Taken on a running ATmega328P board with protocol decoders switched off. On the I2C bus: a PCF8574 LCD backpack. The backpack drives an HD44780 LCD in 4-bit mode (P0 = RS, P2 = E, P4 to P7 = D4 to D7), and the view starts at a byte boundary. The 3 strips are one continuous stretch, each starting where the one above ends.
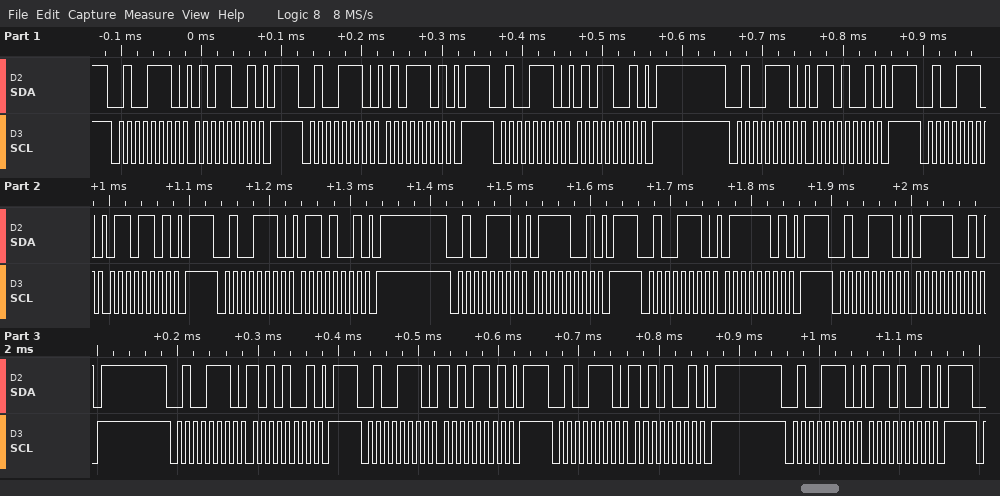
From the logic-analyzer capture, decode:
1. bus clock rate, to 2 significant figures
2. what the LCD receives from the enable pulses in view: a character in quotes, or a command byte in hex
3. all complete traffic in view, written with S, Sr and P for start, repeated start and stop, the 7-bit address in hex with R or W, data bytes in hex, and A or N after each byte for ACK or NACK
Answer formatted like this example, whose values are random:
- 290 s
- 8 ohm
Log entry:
- 100 kHz
- 'V' 'z'
- S 27W A 59 A P S 27W A 5D A P S 27W A 59 A P S 27W A 69 A P S 27W A 6D A P S 27W A 69 A P S 27W A 79 A P S 27W A 7D A P S 27W A 79 A P S 27W A A9 A P S 27W A AD A P S 27W A A9 A P S 27W A 69 A P
